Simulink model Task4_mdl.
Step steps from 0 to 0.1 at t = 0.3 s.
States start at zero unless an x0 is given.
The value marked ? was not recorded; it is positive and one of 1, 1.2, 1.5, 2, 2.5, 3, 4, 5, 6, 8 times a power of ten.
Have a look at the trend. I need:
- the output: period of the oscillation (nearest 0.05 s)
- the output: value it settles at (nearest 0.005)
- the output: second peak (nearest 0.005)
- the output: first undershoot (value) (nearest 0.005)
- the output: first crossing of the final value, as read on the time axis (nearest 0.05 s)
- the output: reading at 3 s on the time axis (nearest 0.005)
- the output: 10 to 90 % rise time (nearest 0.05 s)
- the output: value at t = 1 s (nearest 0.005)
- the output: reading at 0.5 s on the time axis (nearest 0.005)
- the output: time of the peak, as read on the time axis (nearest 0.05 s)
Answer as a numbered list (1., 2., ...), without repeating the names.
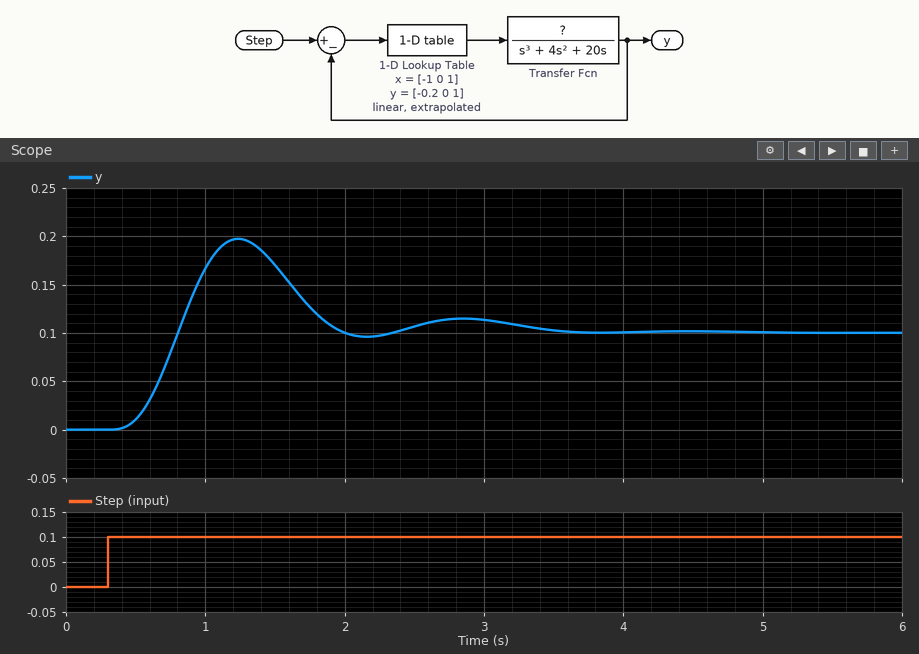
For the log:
1. 1.60 s
2. 0.100
3. 0.115
4. 0.095
5. 0.80 s
6. 0.115
7. 0.30 s
8. 0.165
9. 0.010
10. 1.25 s
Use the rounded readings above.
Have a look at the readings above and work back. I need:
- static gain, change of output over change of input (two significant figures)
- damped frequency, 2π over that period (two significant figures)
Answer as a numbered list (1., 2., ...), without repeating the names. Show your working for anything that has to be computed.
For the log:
1. (0.1 - 0) / (0.1 - 0) = 1.0
2. 2π / 1.6 = 3.9 rad/s
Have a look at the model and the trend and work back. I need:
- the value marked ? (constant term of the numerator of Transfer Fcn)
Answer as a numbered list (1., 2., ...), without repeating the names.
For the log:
1. 100
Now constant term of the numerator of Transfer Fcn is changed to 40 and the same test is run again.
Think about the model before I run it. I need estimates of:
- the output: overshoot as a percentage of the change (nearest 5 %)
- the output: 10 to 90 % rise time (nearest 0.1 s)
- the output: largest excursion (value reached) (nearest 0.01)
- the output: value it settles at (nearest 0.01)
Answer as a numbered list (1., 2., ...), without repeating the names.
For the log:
1. 20 %
2. 0.5 s
3. 0.12
4. 0.10
